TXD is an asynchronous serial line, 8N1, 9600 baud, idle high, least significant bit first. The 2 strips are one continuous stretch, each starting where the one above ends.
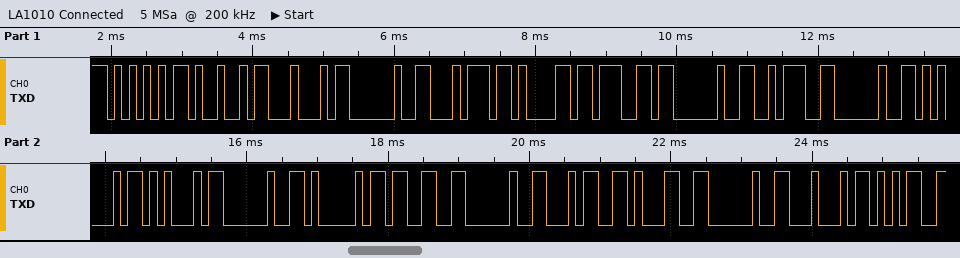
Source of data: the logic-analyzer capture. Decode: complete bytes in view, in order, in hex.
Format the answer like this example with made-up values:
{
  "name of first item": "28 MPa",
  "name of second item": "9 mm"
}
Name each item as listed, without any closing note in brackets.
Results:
{
  "complete bytes in view, in order, in hex": "55 49 44 20 74 61 67 20 3A 20 45 45 20 41 33 20 34 31 20 44 35"
}
